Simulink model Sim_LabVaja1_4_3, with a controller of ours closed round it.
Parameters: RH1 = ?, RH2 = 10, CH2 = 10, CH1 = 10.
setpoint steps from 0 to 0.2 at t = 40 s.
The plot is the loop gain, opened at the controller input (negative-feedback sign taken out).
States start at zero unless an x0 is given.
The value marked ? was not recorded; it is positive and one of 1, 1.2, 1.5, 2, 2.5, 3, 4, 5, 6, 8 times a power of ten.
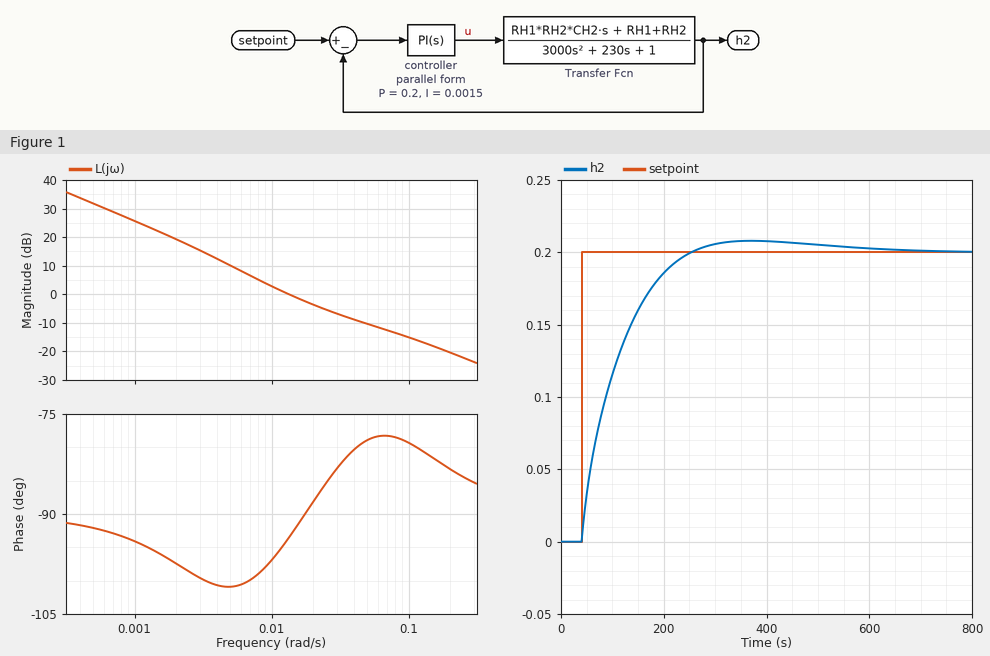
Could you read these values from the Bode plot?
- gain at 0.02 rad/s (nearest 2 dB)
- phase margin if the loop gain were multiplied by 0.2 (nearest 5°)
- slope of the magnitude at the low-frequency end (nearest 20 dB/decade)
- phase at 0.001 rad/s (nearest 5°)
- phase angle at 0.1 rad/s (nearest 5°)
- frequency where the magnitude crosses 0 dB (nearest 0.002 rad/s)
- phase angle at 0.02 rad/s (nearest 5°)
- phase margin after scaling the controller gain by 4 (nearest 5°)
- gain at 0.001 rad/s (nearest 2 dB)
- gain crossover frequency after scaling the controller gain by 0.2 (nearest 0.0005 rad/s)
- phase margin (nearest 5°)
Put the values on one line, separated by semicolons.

-4 dB; 80°; -20 dB/decade; -95°; -80°; 0.014 rad/s; -90°; 100°; 26 dB; 0.0035 rad/s; 85°
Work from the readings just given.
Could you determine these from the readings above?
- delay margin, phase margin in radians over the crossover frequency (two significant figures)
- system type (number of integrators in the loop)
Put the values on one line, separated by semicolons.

110 s; 1
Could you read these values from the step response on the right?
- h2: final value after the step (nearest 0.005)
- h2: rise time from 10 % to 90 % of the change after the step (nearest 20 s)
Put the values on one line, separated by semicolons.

0.200; 140 s
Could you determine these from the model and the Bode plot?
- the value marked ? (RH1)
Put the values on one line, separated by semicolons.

3
